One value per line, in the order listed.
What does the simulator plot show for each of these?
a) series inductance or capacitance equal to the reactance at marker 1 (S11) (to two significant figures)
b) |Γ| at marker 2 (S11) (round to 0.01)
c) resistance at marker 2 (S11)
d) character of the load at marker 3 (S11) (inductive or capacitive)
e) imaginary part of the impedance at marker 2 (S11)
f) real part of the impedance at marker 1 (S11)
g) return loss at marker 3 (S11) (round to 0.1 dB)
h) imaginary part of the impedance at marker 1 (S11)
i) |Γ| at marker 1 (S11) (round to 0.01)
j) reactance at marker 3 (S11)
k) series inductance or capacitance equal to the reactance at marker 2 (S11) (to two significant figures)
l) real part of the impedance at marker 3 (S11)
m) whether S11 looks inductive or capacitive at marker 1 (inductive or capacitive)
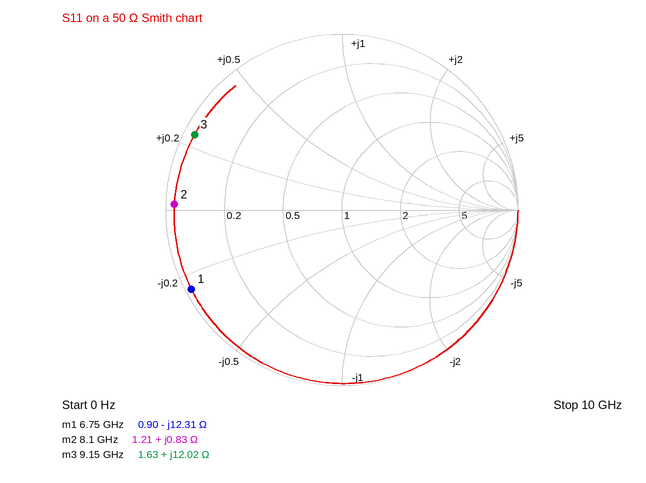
1.9 pF
0.95
1.21 Ω
inductive
+0.83 Ω
0.90 Ω
0.5 dB
-12.31 Ω
0.97
+12.02 Ω
16 pH
1.63 Ω
capacitive
